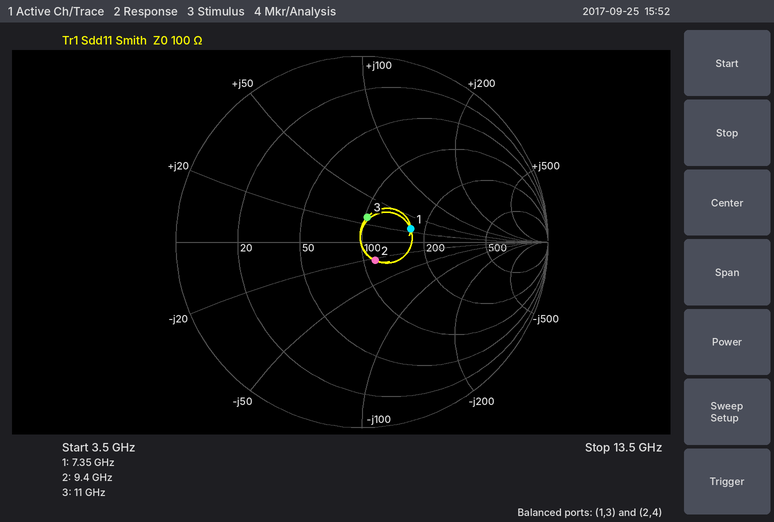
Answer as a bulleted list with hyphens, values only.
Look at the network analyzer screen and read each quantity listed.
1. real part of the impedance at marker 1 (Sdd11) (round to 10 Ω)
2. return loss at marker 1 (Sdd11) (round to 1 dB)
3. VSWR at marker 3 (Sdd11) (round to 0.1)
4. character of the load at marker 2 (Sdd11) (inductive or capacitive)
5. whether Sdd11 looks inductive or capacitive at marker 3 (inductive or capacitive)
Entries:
- 170 Ω
- 11 dB
- 1.3
- capacitive
- inductive
